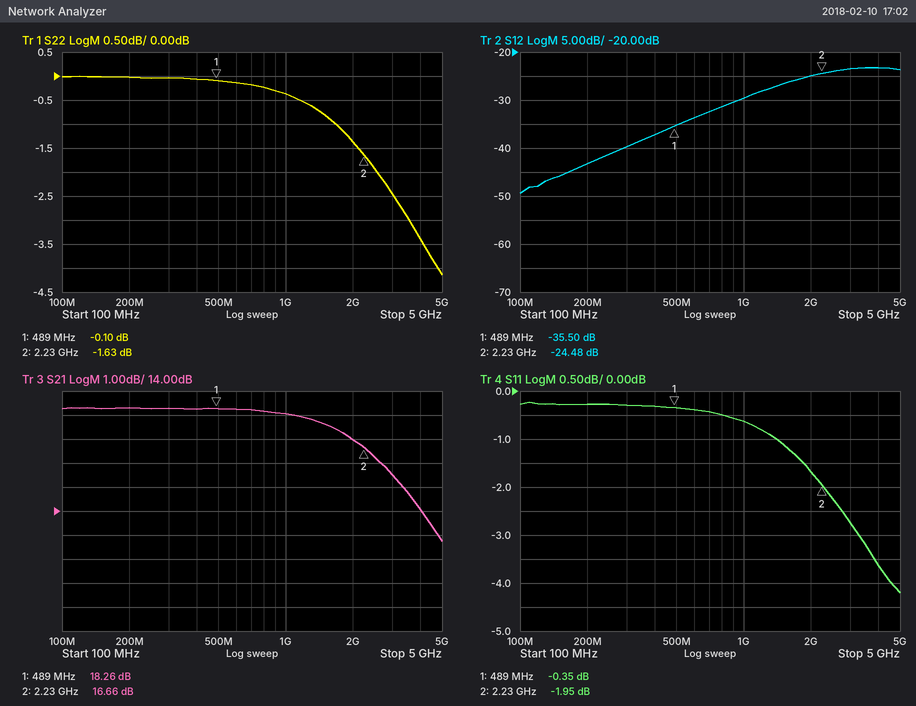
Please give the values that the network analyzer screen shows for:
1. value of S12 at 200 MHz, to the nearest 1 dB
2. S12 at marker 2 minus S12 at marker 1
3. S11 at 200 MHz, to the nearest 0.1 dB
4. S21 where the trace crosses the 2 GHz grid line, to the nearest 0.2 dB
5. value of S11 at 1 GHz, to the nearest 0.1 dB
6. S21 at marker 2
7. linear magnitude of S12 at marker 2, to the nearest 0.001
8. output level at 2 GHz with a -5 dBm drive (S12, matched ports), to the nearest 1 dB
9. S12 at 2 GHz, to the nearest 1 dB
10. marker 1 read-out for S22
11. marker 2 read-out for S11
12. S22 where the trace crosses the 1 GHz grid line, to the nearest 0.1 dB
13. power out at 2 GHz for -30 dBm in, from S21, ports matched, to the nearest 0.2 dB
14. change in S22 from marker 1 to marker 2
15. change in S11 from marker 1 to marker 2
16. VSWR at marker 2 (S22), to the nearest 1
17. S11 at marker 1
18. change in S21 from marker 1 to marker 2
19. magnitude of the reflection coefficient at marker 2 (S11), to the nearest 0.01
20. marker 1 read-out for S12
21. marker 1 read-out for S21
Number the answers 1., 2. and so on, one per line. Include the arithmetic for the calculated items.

1. -43 dB
2. -24.48 − (-35.5) = 11.02 dB
3. -0.3 dB
4. 17.0 dB
5. -0.6 dB
6. 16.66 dB
7. 10^(-24.48/20) ≈ 0.060
8. -5 dBm + (-25 dB) = -30 dBm
9. -25 dB
10. -0.10 dB
11. -1.95 dB
12. -0.4 dB
13. -30 dBm + (17.0 dB) = -13.0 dBm
14. -1.63 − (-0.1) = -1.53 dB
15. -1.95 − (-0.35) = -1.60 dB
16. (1 + 0.8289)/(1 − 0.8289) ≈ 11
17. -0.35 dB
18. 16.66 − (18.26) = -1.60 dB
19. 10^(-1.95/20) ≈ 0.80
20. -35.50 dB
21. 18.26 dB
